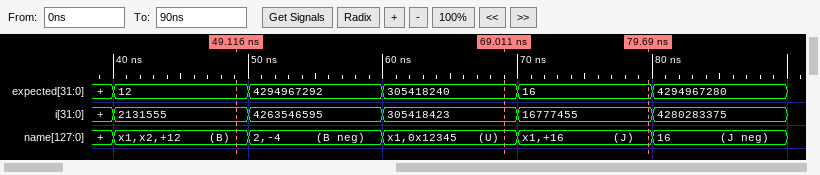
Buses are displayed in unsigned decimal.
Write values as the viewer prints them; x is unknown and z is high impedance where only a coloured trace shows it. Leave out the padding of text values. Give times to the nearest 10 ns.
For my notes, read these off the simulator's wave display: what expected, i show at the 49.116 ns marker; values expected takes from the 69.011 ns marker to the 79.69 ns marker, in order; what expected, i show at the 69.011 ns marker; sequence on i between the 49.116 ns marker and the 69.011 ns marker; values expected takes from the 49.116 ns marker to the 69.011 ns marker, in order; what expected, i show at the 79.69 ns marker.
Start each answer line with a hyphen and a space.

- expected=12, i=2131555
- 305418240, 16
- expected=305418240, i=305418423
- 2131555, 4263546595, 305418423
- 12, 4294967292, 305418240
- expected=16, i=16777455
